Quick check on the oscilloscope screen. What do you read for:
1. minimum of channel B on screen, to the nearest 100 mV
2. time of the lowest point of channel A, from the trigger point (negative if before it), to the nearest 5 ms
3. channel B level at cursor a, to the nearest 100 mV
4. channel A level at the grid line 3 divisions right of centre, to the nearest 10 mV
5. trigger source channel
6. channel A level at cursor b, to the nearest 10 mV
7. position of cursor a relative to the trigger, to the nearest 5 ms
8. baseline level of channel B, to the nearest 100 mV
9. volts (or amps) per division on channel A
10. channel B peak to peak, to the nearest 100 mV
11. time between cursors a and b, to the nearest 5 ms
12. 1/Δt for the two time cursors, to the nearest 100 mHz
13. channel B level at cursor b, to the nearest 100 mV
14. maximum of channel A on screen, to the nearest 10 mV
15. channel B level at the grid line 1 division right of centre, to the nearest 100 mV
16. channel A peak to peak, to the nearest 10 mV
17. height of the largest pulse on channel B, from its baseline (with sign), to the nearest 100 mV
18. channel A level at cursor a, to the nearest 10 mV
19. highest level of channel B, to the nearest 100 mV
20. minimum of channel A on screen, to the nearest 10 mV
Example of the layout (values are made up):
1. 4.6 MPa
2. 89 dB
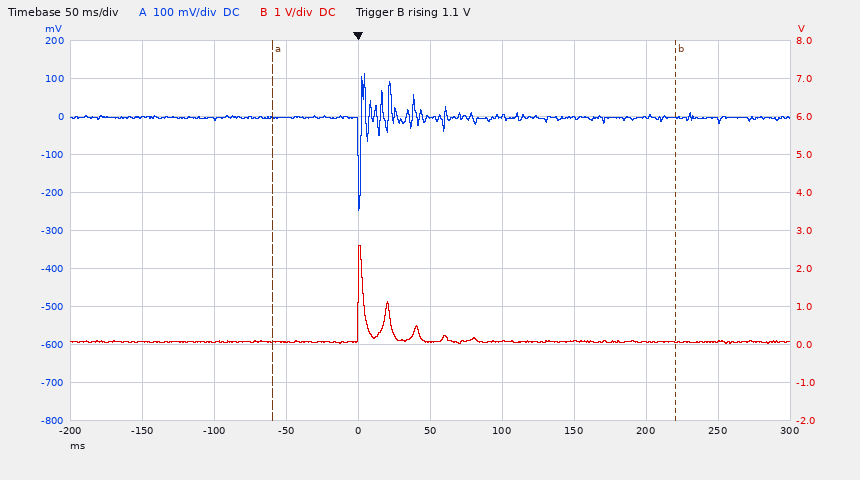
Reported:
1. 0.0 V
2. 0 ms
3. 100 mV
4. 0 mV
5. channel B
6. 0 mV
7. -60 ms
8. 100 mV
9. 100 mV
10. 2.6 V
11. 280 ms
12. 3.6 Hz
13. 100 mV
14. 110 mV
15. 100 mV
16. 360 mV
17. +2.5 V
18. 0 mV
19. 2.6 V
20. -250 mV
